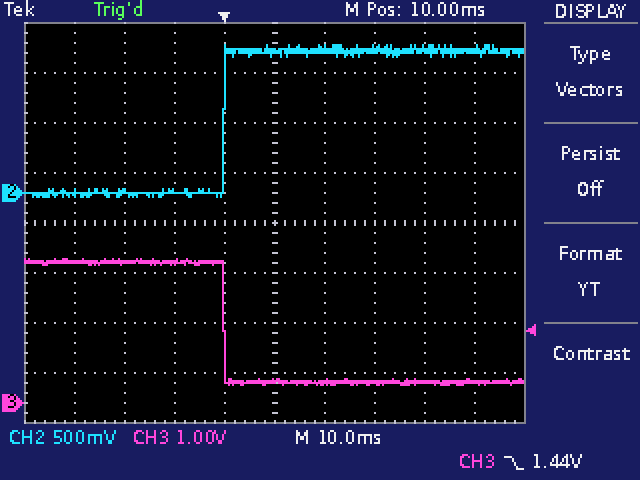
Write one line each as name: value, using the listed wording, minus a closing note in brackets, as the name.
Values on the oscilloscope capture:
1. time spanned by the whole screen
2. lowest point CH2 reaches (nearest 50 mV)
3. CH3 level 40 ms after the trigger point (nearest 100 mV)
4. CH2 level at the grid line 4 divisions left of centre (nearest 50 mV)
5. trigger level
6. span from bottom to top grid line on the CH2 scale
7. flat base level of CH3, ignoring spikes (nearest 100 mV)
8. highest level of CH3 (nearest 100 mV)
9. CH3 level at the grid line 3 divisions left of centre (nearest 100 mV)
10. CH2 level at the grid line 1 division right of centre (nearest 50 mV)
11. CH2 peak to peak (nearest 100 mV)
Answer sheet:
time spanned by the whole screen: 100 ms
lowest point CH2 reaches: -50 mV
CH3 level 40 ms after the trigger point: 400 mV
CH2 level at the grid line 4 divisions left of centre: 0 mV
trigger level: 1.44 V
span from bottom to top grid line on the CH2 scale: 4 V
flat base level of CH3, ignoring spikes: 400 mV
highest level of CH3: 2.9 V
CH3 level at the grid line 3 divisions left of centre: 2.8 V
CH2 level at the grid line 1 division right of centre: 1.45 V
CH2 peak to peak: 1.50 V
